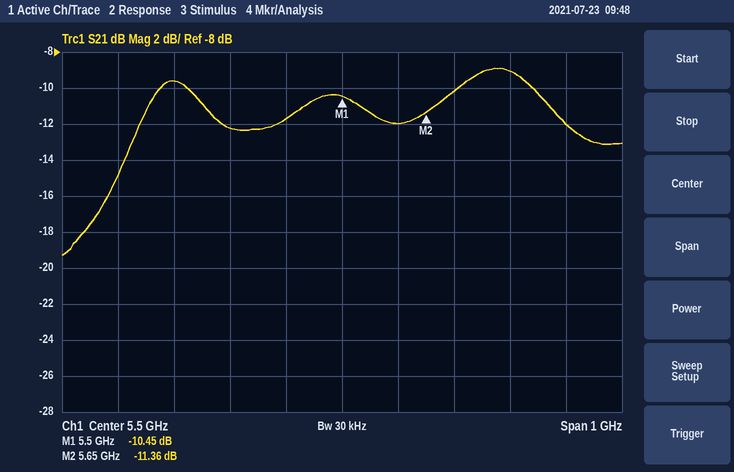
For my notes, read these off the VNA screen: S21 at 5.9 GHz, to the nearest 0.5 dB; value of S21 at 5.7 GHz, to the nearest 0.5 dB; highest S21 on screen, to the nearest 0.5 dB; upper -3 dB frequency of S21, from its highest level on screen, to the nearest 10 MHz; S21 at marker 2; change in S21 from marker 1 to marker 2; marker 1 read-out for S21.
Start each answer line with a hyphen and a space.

- -12.0 dB
- -10.0 dB
- -9.0 dB
- 5.90 GHz
- -11.36 dB
- -0.91 dB
- -10.45 dB
